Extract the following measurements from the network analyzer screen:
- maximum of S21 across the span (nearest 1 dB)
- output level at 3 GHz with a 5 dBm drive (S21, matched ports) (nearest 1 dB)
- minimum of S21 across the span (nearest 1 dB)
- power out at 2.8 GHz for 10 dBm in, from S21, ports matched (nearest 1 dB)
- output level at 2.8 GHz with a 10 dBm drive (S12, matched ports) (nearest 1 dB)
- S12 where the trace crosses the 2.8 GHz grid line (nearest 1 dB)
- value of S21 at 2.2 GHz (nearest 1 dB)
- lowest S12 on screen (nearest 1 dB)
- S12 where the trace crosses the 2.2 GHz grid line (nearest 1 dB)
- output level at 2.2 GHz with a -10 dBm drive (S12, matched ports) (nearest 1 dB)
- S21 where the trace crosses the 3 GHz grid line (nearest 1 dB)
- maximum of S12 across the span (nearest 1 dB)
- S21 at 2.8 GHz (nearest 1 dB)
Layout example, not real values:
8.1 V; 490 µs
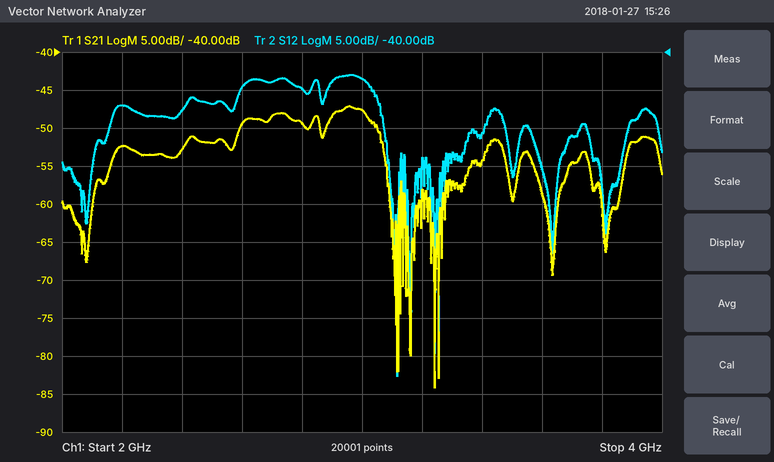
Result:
-47 dB; -43 dBm; -84 dB; -39 dBm; -35 dBm; -45 dB; -52 dB; -83 dB; -47 dB; -57 dBm; -48 dB; -43 dB; -49 dB
